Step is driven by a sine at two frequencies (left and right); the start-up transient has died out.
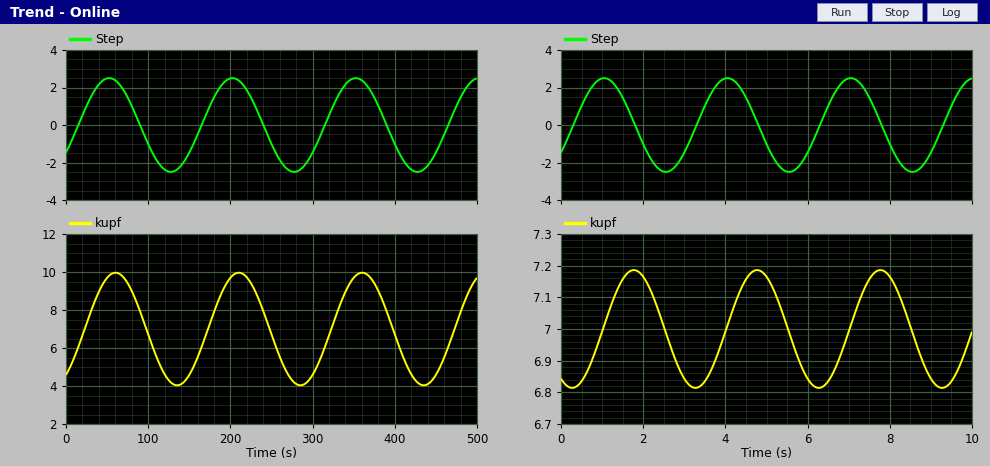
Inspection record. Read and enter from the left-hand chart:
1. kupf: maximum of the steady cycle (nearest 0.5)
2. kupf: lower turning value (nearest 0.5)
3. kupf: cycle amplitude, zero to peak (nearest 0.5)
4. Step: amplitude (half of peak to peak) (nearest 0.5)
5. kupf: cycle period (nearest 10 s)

10.0
4.0
3.0
2.5
150 s
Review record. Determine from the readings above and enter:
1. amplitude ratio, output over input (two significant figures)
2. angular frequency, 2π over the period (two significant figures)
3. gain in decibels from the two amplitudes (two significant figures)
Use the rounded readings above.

1.2
0.042 rad/s
1.6 dB
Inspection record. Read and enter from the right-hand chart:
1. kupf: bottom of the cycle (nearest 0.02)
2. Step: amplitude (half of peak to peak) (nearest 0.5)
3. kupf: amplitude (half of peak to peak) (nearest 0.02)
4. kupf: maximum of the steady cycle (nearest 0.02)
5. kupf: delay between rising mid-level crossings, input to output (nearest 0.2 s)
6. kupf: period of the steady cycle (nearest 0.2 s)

6.82
2.5
0.18
7.18
0.8 s
3.0 s
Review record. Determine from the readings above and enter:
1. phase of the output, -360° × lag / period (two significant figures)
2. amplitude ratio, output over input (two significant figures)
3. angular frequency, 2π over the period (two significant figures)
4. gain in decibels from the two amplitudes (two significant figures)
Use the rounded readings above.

-96°
0.072
2.1 rad/s
-23 dB
